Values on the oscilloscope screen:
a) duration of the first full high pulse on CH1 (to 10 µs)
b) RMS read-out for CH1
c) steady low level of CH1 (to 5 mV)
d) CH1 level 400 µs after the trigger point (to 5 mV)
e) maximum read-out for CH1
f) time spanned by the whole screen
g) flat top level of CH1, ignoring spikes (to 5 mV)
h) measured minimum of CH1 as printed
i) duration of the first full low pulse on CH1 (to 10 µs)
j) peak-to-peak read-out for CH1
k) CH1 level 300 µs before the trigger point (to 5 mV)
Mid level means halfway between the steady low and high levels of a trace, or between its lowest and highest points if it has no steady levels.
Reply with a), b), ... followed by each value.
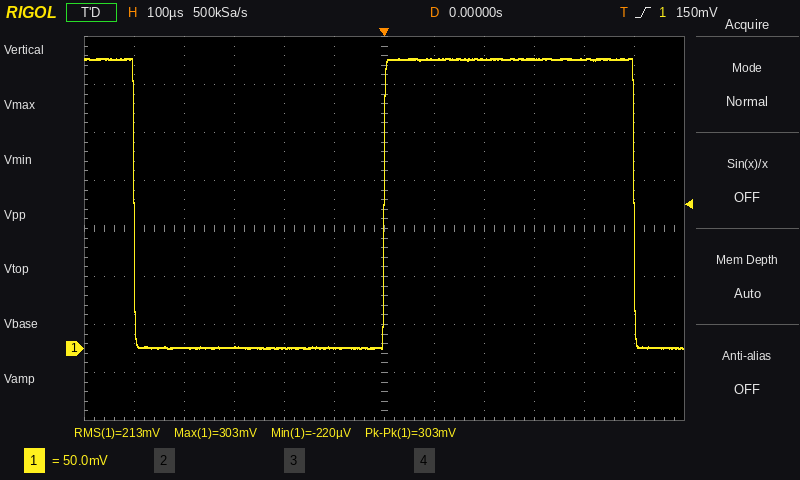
a) 500 µs
b) 213 mV
c) 0 mV
d) 300 mV
e) 303 mV
f) 1.2 ms
g) 300 mV
h) -220 µV
i) 500 µs
j) 303 mV
k) 0 mV
